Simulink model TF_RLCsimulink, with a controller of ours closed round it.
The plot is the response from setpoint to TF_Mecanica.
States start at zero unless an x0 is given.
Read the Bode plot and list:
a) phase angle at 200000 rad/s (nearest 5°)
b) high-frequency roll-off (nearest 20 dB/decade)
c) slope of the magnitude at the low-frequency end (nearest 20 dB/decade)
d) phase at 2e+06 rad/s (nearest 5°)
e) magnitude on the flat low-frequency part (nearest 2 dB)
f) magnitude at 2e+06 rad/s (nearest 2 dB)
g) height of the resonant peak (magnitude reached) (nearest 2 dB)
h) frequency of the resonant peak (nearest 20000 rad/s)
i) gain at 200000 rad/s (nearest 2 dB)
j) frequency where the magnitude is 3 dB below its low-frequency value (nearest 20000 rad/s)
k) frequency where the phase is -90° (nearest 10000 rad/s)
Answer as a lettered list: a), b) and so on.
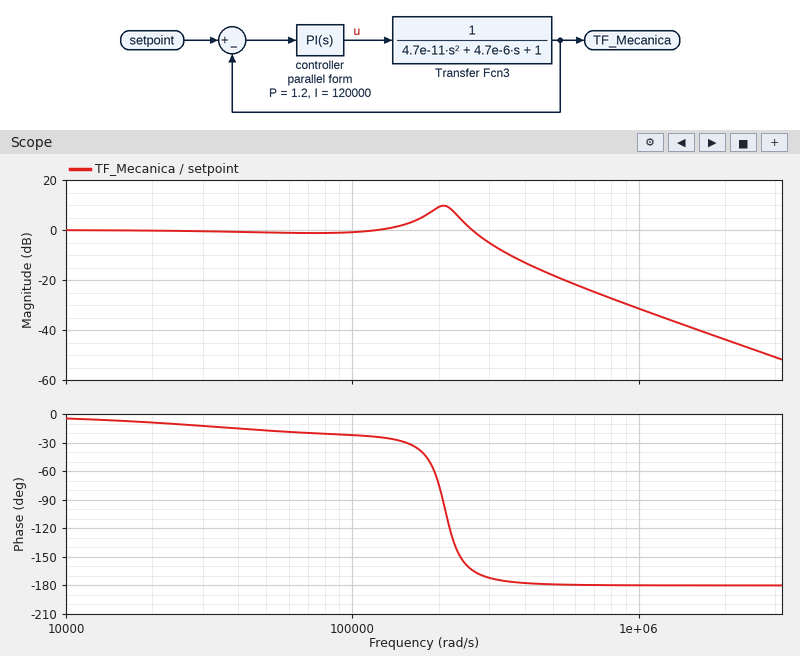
a) -75°
b) -40 dB/decade
c) 0 dB/decade
d) -180°
e) 0 dB
f) -44 dB
g) 10 dB
h) 200000 rad/s
i) 10 dB
j) 280000 rad/s
k) 210000 rad/s
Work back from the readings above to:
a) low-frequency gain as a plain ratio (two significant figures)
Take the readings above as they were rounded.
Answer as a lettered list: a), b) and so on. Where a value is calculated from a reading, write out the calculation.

a) 10^(0 / 20) = 1.0
